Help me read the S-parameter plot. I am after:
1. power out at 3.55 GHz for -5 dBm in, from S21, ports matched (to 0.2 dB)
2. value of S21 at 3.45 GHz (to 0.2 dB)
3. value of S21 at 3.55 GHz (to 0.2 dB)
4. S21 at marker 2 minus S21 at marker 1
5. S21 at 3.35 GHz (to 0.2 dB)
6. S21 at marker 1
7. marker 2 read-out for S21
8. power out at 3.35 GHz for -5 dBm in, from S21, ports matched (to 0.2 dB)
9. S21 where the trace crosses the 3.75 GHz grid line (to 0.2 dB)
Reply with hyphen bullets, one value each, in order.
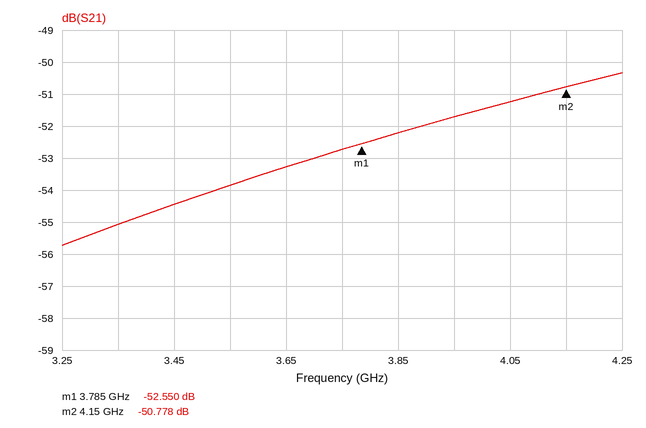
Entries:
- -58.8 dBm
- -54.4 dB
- -53.8 dB
- 1.772 dB
- -55.0 dB
- -52.550 dB
- -50.778 dB
- -60.0 dBm
- -52.8 dB
